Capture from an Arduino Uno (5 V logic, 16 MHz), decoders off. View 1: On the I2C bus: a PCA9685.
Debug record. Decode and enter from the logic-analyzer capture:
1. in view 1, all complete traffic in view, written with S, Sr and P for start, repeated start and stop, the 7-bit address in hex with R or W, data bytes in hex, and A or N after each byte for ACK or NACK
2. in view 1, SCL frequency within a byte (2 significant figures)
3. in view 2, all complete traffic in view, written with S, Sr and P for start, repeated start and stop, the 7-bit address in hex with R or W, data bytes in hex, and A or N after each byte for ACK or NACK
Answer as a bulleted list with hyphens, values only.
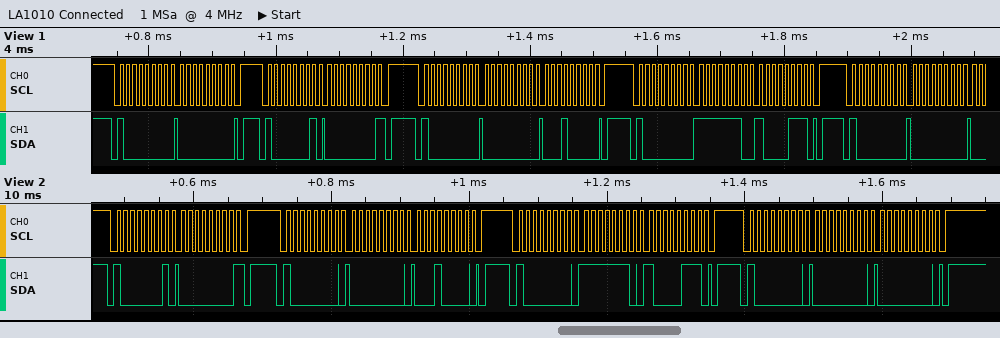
- S 40W A 00 A P S 40R A 00 N P S 40W A 00 A 10 A P S 40W A FE A 87 A P S 40W A 00 A
- 100 kHz
- S 40R A 00 N P S 40W A 00 A 10 A P S 40W A FE A 87 A P S 40W A 00 A 00 A P
